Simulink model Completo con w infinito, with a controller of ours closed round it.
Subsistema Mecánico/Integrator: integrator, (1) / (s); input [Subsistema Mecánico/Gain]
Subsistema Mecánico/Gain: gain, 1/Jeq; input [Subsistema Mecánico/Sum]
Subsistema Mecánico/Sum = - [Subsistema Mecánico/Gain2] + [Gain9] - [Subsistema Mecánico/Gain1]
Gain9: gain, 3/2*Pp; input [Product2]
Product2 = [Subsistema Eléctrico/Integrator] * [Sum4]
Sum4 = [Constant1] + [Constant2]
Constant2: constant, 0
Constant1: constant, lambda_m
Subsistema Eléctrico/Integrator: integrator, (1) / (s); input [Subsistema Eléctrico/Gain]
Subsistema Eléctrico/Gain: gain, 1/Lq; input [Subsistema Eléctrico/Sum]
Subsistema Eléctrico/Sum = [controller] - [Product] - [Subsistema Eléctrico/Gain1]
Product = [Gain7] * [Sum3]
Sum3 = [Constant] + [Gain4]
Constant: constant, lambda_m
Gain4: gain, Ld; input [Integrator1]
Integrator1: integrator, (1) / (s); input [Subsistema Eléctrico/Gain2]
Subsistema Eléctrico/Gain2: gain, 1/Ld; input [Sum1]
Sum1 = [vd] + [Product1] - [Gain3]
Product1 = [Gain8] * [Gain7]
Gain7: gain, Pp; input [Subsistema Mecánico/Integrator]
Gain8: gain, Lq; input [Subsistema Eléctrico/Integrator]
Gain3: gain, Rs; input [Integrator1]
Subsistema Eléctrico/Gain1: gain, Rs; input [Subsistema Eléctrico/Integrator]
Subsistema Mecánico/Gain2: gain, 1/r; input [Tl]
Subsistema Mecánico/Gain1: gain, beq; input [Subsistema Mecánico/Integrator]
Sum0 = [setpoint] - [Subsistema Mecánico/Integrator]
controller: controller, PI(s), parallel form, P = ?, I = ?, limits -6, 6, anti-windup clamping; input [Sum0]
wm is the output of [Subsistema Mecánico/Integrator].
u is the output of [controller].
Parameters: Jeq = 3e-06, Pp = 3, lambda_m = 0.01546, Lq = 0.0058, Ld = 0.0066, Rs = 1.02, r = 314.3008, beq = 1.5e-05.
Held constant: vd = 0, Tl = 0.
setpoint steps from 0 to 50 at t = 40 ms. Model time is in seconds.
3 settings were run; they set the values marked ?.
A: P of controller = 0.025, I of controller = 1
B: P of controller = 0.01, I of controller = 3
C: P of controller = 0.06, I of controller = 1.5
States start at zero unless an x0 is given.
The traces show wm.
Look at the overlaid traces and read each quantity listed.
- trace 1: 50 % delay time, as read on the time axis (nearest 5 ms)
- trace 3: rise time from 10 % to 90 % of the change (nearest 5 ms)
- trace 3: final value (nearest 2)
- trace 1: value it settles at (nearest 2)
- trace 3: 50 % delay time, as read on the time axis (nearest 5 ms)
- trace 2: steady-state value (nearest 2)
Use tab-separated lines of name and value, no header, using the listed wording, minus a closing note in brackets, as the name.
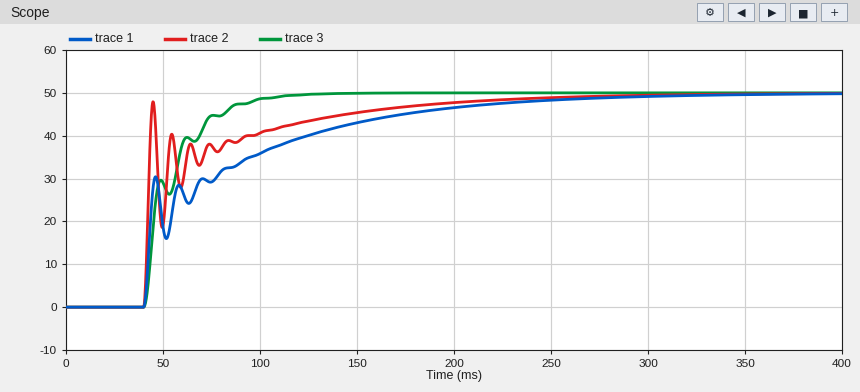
trace 1: 50 % delay time, as read on the time axis	45 ms
trace 3: rise time from 10 % to 90 % of the change	40 ms
trace 3: final value	50
trace 1: value it settles at	50
trace 3: 50 % delay time, as read on the time axis	45 ms
trace 2: steady-state value	50
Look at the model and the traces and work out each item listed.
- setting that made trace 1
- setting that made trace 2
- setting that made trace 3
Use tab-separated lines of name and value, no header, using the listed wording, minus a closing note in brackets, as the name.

setting that made trace 1	A
setting that made trace 2	C
setting that made trace 3	B
